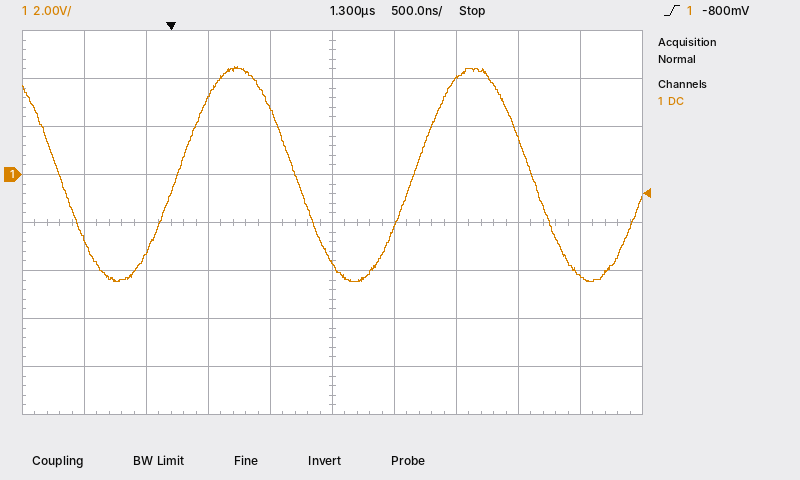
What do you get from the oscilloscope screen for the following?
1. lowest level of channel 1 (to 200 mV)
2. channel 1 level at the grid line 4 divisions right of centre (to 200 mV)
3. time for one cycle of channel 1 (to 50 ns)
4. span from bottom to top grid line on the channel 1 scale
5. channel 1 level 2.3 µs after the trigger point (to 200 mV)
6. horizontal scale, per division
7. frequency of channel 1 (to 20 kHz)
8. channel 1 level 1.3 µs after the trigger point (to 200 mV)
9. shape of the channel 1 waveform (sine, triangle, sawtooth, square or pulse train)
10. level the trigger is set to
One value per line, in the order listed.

-4.4 V
-4.2 V
1.90 µs
16 V
4.0 V
500 ns
520 kHz
-3.6 V
sine
-800 mV
